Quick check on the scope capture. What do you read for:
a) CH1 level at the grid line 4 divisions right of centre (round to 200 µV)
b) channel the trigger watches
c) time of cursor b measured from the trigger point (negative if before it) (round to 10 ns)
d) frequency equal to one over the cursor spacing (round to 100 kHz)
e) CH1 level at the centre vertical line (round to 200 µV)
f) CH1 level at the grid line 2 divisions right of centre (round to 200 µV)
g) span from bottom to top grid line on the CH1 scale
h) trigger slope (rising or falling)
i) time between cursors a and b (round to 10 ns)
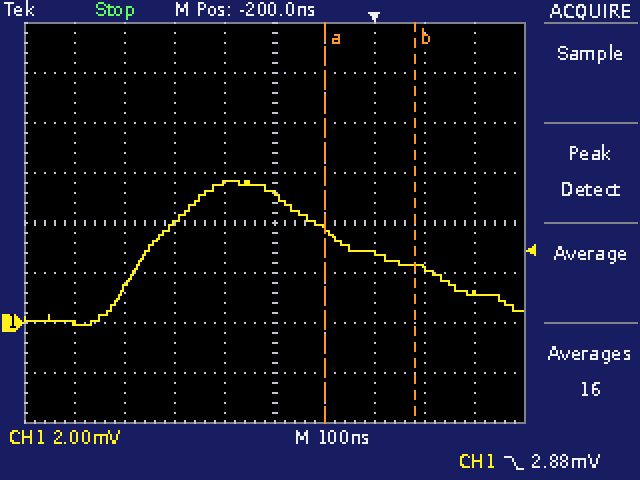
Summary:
1.2 mV
CH1
+80 ns
5.6 MHz
5.2 mV
2.8 mV
16 mV
falling
180 ns
